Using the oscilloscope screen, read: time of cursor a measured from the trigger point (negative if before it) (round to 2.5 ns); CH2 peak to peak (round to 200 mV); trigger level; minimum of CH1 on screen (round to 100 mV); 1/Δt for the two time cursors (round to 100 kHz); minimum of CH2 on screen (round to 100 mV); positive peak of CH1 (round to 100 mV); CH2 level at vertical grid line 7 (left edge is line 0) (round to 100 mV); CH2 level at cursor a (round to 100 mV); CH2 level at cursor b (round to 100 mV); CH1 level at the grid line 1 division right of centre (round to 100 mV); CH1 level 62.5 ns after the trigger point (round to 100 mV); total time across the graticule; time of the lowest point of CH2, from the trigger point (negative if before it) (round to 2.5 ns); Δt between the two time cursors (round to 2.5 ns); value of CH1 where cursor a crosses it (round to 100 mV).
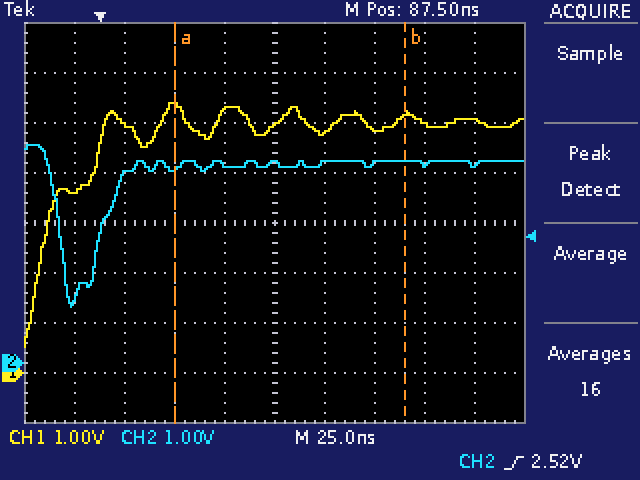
+37.5 ns
3.2 V
2.52 V
500 mV
8.7 MHz
1.1 V
5.4 V
4.0 V
3.9 V
4.0 V
4.8 V
5.2 V
250 ns
-15.0 ns
115.0 ns
5.3 V
